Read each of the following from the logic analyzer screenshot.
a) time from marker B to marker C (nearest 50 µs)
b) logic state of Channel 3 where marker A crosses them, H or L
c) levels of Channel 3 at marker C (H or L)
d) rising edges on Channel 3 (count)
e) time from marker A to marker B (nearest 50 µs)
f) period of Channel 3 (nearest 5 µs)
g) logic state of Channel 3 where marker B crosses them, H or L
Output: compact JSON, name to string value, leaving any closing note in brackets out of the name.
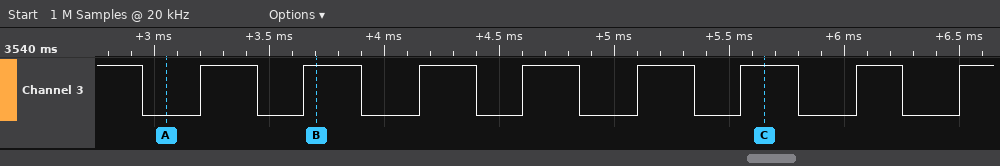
{"time from marker B to marker C": "1950 µs", "logic state of Channel 3 where marker A crosses them, H or L": "Channel 3=L", "levels of Channel 3 at marker C": "Channel 3=H", "rising edges on Channel 3": "8", "time from marker A to marker B": "650 µs", "period of Channel 3": "470 µs", "logic state of Channel 3 where marker B crosses them, H or L": "Channel 3=H"}
